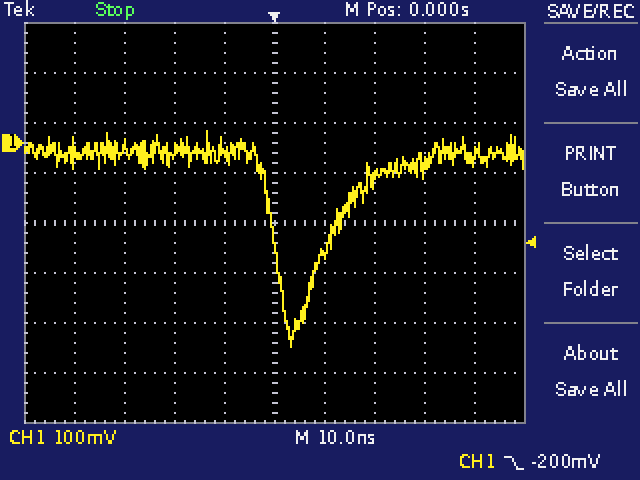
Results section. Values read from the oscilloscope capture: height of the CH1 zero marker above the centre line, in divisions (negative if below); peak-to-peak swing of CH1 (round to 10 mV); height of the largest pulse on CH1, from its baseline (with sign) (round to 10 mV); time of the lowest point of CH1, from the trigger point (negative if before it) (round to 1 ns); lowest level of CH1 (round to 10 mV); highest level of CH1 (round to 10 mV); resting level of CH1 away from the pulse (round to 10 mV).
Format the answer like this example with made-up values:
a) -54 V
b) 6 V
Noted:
a) +1.6 div
b) 430 mV
c) -390 mV
d) +3 ns
e) -410 mV
f) 20 mV
g) -20 mV
